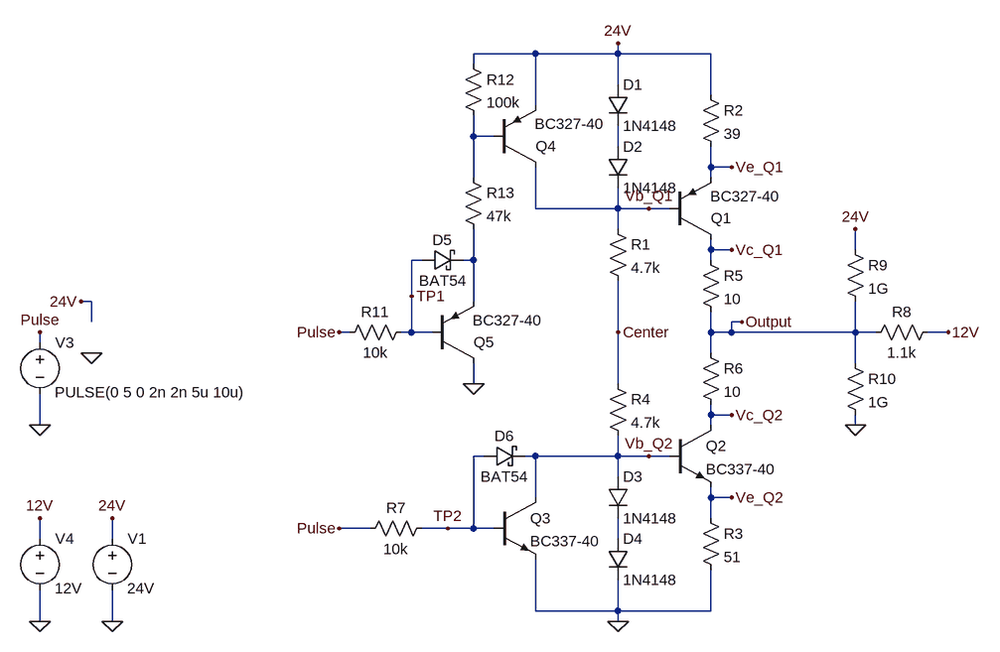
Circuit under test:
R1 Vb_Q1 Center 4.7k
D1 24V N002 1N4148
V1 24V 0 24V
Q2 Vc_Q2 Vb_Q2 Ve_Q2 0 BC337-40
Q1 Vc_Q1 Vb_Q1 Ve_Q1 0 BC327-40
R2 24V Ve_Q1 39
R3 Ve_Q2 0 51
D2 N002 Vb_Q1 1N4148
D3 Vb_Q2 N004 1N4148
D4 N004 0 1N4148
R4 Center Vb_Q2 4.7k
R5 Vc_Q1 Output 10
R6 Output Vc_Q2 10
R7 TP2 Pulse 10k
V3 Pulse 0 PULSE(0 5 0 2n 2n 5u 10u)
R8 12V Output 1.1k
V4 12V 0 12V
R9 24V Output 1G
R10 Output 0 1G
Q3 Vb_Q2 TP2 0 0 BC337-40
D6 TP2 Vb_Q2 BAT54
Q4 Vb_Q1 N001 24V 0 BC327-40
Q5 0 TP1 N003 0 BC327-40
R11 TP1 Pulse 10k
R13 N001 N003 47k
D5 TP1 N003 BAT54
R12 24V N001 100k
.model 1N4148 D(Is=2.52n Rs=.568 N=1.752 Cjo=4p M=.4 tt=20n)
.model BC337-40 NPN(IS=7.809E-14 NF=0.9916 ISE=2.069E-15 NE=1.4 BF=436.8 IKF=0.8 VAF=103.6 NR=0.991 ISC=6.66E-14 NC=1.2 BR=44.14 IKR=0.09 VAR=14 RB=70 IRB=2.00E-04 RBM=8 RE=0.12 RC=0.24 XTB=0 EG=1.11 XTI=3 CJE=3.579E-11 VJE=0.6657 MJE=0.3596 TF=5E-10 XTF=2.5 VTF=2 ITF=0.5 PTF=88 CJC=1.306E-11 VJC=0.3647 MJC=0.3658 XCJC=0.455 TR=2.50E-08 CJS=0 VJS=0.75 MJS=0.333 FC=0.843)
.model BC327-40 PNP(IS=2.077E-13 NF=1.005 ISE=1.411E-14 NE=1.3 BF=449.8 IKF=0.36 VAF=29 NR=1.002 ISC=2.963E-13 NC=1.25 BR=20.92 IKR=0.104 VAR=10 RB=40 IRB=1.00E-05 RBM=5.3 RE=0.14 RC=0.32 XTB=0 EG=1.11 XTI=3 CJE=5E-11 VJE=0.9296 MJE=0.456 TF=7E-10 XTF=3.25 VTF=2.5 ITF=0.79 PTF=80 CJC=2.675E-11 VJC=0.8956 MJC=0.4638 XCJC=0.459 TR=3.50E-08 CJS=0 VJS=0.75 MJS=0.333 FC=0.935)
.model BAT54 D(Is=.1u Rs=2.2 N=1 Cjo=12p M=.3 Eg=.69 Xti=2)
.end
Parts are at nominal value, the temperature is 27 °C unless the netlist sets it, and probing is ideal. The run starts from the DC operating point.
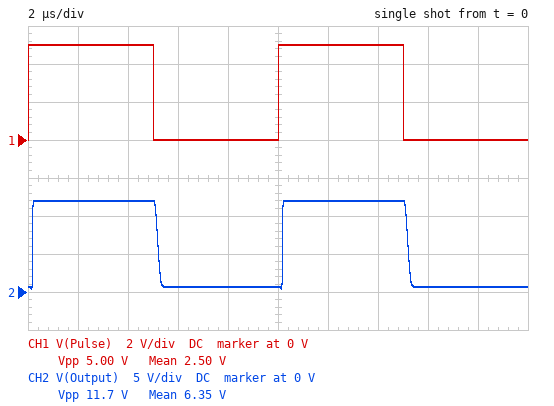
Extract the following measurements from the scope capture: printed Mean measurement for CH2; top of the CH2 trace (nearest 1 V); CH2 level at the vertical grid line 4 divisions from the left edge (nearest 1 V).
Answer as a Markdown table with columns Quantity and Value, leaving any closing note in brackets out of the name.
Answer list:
| Quantity | Value |
|---|---|
| printed Mean measurement for CH2 | 6.35 V |
| top of the CH2 trace | 12 V |
| CH2 level at the vertical grid line 4 divisions from the left edge | 1 V |
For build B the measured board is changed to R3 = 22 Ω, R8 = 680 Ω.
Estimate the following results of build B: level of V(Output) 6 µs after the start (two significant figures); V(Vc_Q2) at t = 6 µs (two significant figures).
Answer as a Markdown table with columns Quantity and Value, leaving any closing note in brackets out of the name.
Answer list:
| Quantity | Value |
|---|---|
| level of V(Output) 6 µs after the start | 600 mV |
| V(Vc_Q2) at t = 6 µs | 430 mV |
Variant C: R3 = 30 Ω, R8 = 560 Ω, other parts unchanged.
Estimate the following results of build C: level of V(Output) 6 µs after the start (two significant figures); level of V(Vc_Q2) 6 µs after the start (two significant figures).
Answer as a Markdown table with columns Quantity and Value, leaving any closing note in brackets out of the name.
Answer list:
| Quantity | Value |
|---|---|
| level of V(Output) 6 µs after the start | 1.4 V |
| level of V(Vc_Q2) 6 µs after the start | 1.2 V |
